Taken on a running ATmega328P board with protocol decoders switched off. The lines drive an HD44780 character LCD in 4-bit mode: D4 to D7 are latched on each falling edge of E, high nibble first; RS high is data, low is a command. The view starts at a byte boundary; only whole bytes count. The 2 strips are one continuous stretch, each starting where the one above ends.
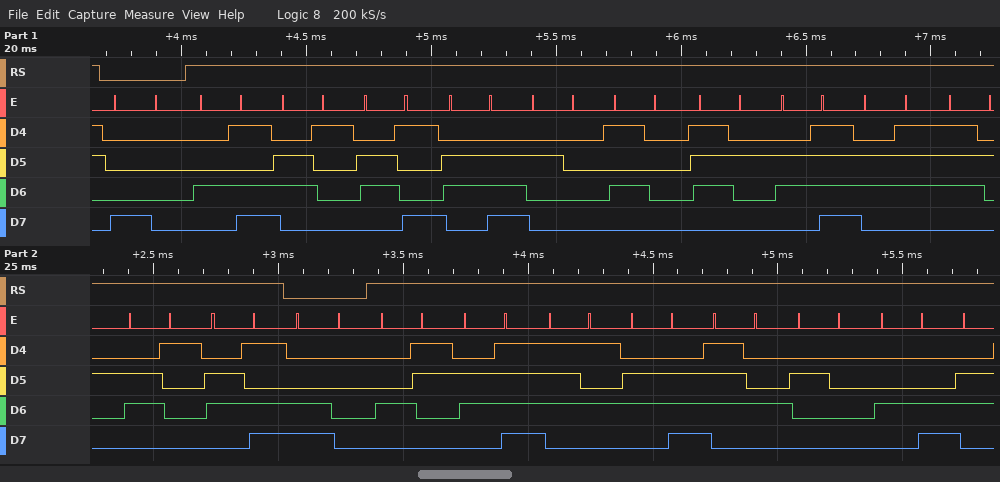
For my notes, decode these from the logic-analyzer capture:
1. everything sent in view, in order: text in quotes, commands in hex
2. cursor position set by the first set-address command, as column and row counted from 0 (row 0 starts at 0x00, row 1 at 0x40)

0x80 "Main Program" 0xC0 "Count L"
column 0, row 0
